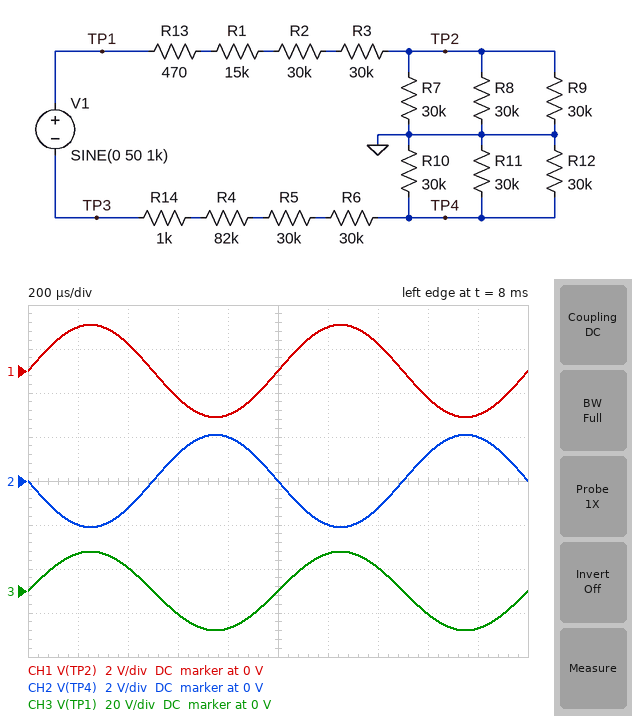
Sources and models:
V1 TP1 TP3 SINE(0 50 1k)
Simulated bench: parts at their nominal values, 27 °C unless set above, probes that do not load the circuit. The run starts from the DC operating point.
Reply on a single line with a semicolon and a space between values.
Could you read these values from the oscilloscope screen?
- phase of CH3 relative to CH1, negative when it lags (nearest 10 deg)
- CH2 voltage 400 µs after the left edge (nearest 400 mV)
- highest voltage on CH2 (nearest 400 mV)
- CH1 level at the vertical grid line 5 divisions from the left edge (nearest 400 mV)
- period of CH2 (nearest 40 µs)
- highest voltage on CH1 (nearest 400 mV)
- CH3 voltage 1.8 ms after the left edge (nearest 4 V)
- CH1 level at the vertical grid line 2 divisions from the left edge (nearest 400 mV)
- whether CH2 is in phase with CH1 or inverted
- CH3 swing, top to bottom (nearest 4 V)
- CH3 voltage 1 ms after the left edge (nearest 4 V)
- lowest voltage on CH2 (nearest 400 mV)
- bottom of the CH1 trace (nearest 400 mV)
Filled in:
0 deg; -1.2 V; 2.0 V; 0 V; 1.00 ms; 2.0 V; -16 V; 1.2 V; inverted; 36 V; 0 V; -2.0 V; -2.0 V
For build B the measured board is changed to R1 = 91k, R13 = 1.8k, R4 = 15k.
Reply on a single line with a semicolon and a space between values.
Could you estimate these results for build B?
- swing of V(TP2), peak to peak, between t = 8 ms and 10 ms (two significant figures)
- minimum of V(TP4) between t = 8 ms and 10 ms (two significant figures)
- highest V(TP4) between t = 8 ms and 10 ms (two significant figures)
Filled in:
4.0 V; -2.0 V; 2.0 V
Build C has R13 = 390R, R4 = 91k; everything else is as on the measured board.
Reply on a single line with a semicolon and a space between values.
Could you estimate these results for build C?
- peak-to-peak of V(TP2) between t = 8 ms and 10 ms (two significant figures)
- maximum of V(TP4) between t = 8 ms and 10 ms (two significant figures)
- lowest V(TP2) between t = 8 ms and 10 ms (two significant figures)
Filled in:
4.0 V; 2.0 V; -2.0 V
